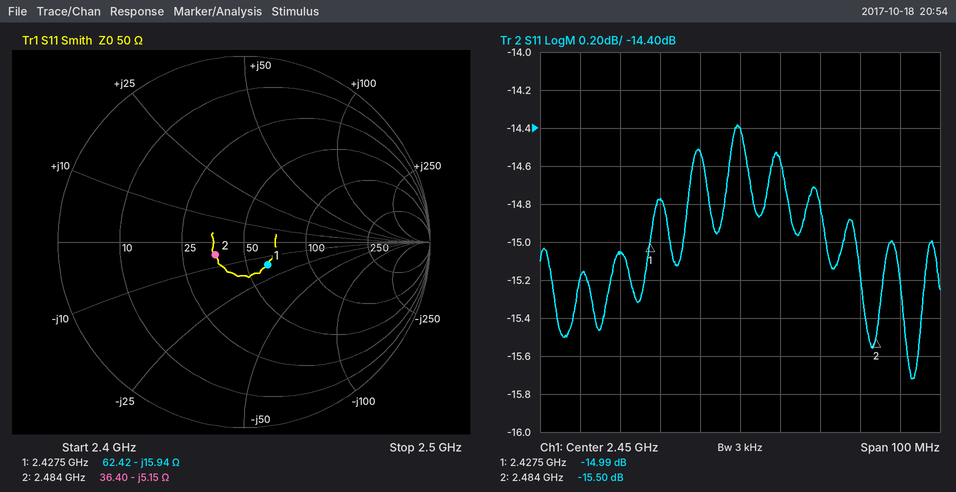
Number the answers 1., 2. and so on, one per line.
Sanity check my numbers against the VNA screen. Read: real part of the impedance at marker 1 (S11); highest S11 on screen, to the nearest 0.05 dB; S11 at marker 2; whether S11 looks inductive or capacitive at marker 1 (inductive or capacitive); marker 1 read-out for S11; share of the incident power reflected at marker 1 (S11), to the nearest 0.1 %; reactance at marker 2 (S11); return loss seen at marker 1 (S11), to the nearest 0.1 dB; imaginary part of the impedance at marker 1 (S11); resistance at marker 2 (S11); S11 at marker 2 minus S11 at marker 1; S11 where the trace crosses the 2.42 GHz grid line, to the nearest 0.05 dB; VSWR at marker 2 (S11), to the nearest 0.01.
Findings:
1. 62.42 Ω
2. -14.40 dB
3. -15.50 dB
4. capacitive
5. -14.99 dB
6. 3.2 %
7. -5.15 Ω
8. 15.0 dB
9. -15.94 Ω
10. 36.40 Ω
11. -0.51 dB
12. -15.05 dB
13. 1.40
